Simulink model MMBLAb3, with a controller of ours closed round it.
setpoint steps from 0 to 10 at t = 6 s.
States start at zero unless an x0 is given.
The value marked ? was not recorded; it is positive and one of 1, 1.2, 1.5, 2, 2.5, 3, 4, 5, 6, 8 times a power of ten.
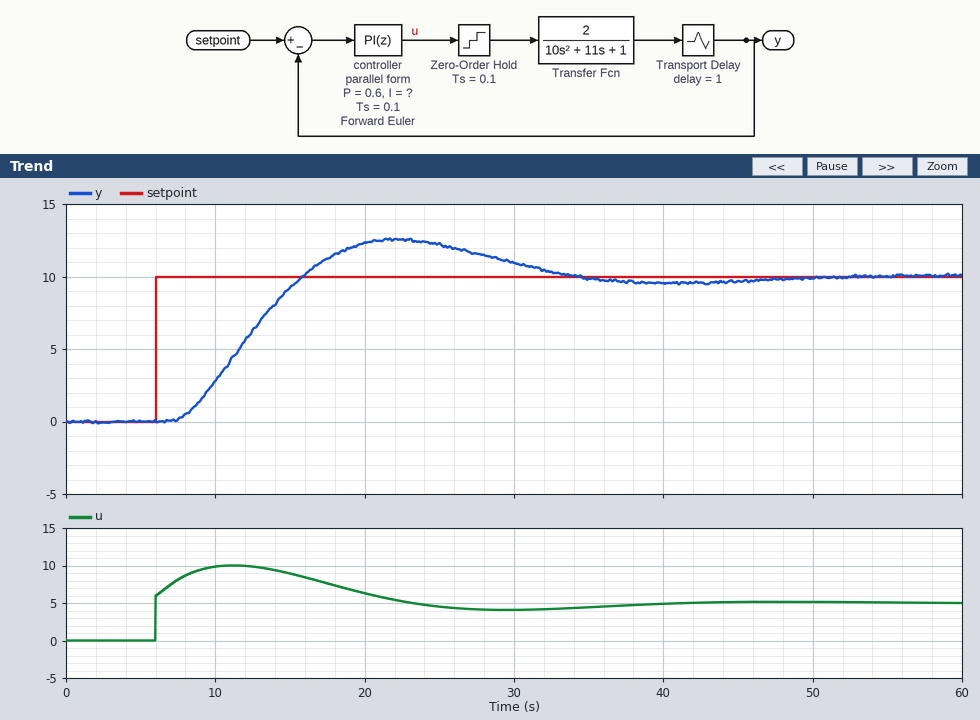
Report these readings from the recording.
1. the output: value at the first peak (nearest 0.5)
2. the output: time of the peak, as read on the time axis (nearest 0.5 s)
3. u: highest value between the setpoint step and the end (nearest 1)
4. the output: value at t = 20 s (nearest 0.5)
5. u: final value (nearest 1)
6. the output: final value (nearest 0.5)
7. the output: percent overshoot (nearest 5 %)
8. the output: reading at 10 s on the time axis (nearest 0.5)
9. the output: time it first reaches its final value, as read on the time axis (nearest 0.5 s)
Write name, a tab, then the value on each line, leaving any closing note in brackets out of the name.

the output: value at the first peak	12.5
the output: time of the peak, as read on the time axis	22.0 s
u: highest value between the setpoint step and the end	10
the output: value at t = 20 s	12.5
u: final value	5
the output: final value	10.0
the output: percent overshoot	25 %
the output: reading at 10 s on the time axis	3.0
the output: time it first reaches its final value, as read on the time axis	16.0 s
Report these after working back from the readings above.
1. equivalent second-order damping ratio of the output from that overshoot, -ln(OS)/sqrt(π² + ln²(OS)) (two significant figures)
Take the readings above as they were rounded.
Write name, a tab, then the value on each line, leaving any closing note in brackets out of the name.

equivalent second-order damping ratio of the output from that overshoot, -ln(OS)/sqrt(π² + ln²(OS))	0.40
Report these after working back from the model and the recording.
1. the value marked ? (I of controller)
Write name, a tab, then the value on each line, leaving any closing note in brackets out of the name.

the value marked ?	0.15
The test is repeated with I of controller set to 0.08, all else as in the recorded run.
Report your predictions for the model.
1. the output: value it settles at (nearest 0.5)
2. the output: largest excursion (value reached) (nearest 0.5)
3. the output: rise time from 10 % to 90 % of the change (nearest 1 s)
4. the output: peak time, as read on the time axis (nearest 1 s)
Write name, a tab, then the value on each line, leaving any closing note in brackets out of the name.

the output: value it settles at	10.0
the output: largest excursion (value reached)	10.5
the output: rise time from 10 % to 90 % of the change	10 s
the output: peak time, as read on the time axis	29 s
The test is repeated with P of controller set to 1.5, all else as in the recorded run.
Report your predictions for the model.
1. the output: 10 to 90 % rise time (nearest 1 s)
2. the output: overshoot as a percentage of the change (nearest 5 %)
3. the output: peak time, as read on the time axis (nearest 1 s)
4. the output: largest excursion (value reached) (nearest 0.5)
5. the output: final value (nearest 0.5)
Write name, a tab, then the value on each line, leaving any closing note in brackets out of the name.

the output: 10 to 90 % rise time	4 s
the output: overshoot as a percentage of the change	10 %
the output: peak time, as read on the time axis	15 s
the output: largest excursion (value reached)	11.0
the output: final value	10.0
